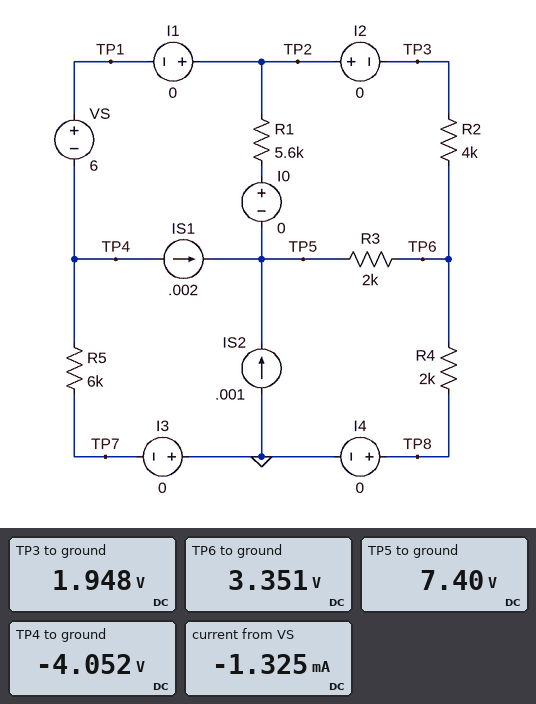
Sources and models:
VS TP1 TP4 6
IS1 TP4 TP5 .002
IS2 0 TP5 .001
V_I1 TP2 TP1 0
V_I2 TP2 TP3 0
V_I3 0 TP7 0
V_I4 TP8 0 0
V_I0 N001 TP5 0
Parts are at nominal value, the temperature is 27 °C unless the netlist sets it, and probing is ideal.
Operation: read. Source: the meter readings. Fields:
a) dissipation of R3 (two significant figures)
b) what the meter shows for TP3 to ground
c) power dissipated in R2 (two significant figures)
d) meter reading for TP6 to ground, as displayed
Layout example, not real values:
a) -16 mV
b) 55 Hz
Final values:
a) 8.2 mW
b) 1.948 V
c) 490 µW
d) 3.351 V
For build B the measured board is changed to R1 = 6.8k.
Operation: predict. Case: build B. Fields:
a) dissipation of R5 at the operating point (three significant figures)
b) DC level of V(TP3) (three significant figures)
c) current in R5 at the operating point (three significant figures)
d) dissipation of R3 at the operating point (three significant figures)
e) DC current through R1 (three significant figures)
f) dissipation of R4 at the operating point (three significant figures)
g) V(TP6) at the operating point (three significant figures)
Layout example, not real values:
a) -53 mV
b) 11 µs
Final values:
a) 3.02 mW
b) 1.74 V
c) 709 µA
d) 9.06 mW
e) 872 µA
f) 5.84 mW
g) 3.42 V
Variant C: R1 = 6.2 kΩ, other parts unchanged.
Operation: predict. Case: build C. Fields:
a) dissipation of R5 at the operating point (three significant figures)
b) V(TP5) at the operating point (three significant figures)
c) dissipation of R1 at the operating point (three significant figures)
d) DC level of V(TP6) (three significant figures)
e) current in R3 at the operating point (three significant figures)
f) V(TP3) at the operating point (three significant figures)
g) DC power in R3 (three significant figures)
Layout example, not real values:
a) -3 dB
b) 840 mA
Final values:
a) 2.88 mW
b) 7.55 V
c) 5.25 mW
d) 3.39 V
e) 2.08 mA
f) 1.84 V
g) 8.65 mW
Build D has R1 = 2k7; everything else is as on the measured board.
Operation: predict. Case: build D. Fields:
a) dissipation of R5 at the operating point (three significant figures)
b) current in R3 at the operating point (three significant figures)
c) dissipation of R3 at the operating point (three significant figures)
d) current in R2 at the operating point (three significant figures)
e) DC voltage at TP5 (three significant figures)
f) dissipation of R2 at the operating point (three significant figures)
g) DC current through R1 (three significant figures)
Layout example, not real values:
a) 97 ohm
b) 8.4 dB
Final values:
a) 1.80 mW
b) 1.64 mA
c) 5.40 mW
d) 95.0 µA
e) 6.38 V
f) 36.1 µW
g) 1.36 mA
